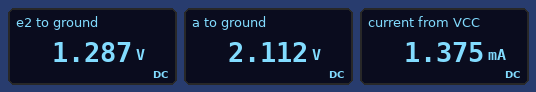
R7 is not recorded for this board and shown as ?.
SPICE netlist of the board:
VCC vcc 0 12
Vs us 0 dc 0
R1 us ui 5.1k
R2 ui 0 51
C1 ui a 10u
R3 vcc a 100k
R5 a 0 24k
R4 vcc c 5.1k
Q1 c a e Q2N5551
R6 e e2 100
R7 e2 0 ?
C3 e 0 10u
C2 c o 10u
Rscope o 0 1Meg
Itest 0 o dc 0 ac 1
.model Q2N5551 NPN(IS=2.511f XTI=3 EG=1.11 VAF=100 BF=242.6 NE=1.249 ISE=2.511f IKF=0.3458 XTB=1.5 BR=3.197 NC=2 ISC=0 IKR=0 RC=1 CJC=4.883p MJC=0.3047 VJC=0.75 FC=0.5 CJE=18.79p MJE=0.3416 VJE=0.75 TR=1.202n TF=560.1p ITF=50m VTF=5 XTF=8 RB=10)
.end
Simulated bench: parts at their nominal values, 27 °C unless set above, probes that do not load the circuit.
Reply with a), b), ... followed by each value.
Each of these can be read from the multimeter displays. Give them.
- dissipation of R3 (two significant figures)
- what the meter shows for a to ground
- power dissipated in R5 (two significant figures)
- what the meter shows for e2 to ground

a) 980 µW
b) 2.112 V
c) 190 µW
d) 1.287 V
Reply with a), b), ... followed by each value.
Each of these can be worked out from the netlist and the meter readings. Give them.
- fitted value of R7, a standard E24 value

a) 1 kΩ
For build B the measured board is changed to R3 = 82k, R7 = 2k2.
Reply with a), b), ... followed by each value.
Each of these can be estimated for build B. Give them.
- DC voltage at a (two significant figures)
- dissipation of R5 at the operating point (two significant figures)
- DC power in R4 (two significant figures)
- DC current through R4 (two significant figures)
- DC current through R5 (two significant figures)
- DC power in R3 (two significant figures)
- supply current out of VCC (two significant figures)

a) 2.6 V
b) 280 µW
c) 3.4 mW
d) 820 µA
e) 110 µA
f) 1.1 mW
g) 930 µA
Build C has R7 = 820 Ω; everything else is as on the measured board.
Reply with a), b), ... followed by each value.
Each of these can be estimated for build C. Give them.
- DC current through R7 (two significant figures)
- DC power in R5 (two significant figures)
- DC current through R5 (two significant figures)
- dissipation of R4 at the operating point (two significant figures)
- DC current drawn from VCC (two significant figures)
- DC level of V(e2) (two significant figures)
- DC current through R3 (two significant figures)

a) 1.5 mA
b) 180 µW
c) 87 µA
d) 11 mW
e) 1.6 mA
f) 1.2 V
g) 99 µA
